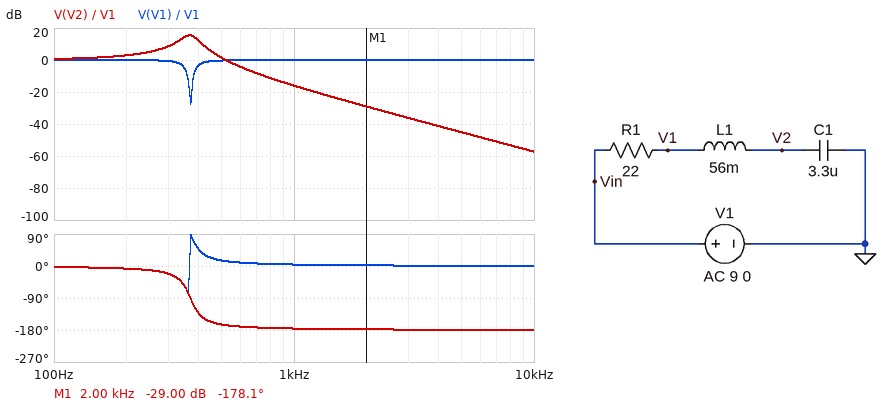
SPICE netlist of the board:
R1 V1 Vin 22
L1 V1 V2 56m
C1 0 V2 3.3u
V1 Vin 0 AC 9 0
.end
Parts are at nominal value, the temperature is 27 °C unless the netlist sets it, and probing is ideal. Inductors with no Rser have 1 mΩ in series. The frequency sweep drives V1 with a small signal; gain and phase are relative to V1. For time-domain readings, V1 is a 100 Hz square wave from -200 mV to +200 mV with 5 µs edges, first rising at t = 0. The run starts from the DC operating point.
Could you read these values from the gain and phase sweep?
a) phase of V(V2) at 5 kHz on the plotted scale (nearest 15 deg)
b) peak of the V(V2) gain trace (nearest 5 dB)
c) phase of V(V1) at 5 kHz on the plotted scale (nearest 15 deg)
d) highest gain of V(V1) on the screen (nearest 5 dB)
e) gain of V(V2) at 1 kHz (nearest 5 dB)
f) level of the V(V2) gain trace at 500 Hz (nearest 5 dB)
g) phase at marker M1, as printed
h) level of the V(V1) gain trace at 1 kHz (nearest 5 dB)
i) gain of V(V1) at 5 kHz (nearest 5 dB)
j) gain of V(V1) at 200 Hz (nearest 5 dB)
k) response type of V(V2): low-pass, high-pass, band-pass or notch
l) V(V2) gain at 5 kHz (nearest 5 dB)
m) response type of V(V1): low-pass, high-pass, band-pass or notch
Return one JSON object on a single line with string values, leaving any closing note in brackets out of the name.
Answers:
{"phase of V(V2) at 5 kHz on the plotted scale": "-180 deg", "peak of the V(V2) gain trace": "15 dB", "phase of V(V1) at 5 kHz on the plotted scale": "0 deg", "highest gain of V(V1) on the screen": "0 dB", "gain of V(V2) at 1 kHz": "-15 dB", "level of the V(V2) gain trace at 500 Hz": "0 dB", "phase at marker M1, as printed": "-178.1 deg", "level of the V(V1) gain trace at 1 kHz": "0 dB", "gain of V(V1) at 5 kHz": "0 dB", "gain of V(V1) at 200 Hz": "0 dB", "response type of V(V2): low-pass, high-pass, band-pass or notch": "low-pass", "V(V2) gain at 5 kHz": "-45 dB", "response type of V(V1): low-pass, high-pass, band-pass or notch": "notch"}
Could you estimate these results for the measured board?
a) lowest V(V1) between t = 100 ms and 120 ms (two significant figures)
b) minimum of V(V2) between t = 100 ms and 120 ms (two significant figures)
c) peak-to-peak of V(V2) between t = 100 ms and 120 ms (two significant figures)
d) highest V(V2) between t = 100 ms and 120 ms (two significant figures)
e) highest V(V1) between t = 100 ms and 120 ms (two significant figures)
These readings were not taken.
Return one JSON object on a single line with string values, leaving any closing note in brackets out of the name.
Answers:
{"lowest V(V1) between t = 100 ms and 120 ms": "-240 mV", "minimum of V(V2) between t = 100 ms and 120 ms": "-450 mV", "peak-to-peak of V(V2) between t = 100 ms and 120 ms": "900 mV", "highest V(V2) between t = 100 ms and 120 ms": "450 mV", "highest V(V1) between t = 100 ms and 120 ms": "240 mV"}
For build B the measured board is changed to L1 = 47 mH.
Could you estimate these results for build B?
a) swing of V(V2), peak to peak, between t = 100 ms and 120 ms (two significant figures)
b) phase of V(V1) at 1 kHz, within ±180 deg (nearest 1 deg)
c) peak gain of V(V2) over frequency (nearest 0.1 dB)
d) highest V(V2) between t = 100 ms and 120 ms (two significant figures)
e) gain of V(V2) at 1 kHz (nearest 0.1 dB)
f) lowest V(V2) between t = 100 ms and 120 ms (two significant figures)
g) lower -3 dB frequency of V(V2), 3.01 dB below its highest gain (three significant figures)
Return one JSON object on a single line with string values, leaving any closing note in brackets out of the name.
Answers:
{"swing of V(V2), peak to peak, between t = 100 ms and 120 ms": "860 mV", "phase of V(V1) at 1 kHz, within ±180 deg": "5 deg", "peak gain of V(V2) over frequency": "14.7 dB", "highest V(V2) between t = 100 ms and 120 ms": "430 mV", "gain of V(V2) at 1 kHz": "-14.2 dB", "lowest V(V2) between t = 100 ms and 120 ms": "-430 mV", "lower -3 dB frequency of V(V2), 3.01 dB below its highest gain": "361 Hz"}
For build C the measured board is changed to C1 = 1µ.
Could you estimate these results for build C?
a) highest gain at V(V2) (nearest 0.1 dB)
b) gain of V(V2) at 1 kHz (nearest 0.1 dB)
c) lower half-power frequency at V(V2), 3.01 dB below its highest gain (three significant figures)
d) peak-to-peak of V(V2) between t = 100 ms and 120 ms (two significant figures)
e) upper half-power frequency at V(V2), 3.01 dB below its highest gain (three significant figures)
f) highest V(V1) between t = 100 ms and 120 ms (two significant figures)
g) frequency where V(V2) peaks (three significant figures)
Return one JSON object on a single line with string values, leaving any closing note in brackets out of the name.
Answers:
{"highest gain at V(V2)": "20.6 dB", "gain of V(V2) at 1 kHz": "-1.7 dB", "lower half-power frequency at V(V2), 3.01 dB below its highest gain": "639 Hz", "peak-to-peak of V(V2) between t = 100 ms and 120 ms": "1.2 V", "upper half-power frequency at V(V2), 3.01 dB below its highest gain": "702 Hz", "highest V(V1) between t = 100 ms and 120 ms": "240 mV", "frequency where V(V2) peaks": "671 Hz"}
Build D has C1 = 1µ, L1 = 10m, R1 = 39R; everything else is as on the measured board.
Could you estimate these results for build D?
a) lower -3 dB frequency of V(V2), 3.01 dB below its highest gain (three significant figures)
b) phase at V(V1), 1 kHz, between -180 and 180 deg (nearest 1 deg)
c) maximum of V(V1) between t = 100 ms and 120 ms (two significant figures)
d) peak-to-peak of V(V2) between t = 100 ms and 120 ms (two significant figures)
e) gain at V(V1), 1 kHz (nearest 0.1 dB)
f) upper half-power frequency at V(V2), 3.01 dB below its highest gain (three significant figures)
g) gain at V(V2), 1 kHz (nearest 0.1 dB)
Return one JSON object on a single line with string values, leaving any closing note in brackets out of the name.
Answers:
{"lower -3 dB frequency of V(V2), 3.01 dB below its highest gain": "1.17 kHz", "phase at V(V1), 1 kHz, between -180 and 180 deg": "-22 deg", "maximum of V(V1) between t = 100 ms and 120 ms": "260 mV", "peak-to-peak of V(V2) between t = 100 ms and 120 ms": "830 mV", "gain at V(V1), 1 kHz": "-0.7 dB", "upper half-power frequency at V(V2), 3.01 dB below its highest gain": "1.82 kHz", "gain at V(V2), 1 kHz": "3.7 dB"}
